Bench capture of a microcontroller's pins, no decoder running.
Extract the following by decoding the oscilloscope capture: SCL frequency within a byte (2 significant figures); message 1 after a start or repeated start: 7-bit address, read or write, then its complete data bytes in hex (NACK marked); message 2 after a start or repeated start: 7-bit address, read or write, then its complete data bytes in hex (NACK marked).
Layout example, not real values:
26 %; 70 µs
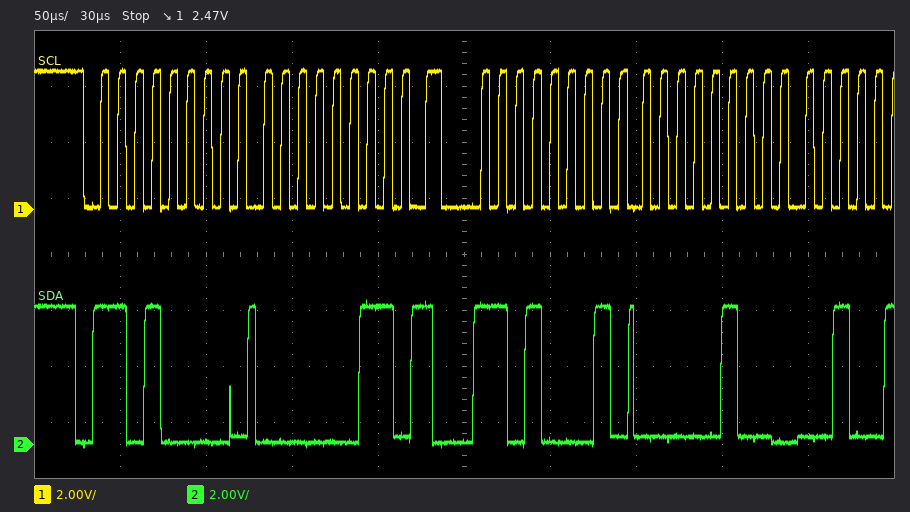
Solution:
100 kHz; 0x68 write: 03; 0x68 read: 04
